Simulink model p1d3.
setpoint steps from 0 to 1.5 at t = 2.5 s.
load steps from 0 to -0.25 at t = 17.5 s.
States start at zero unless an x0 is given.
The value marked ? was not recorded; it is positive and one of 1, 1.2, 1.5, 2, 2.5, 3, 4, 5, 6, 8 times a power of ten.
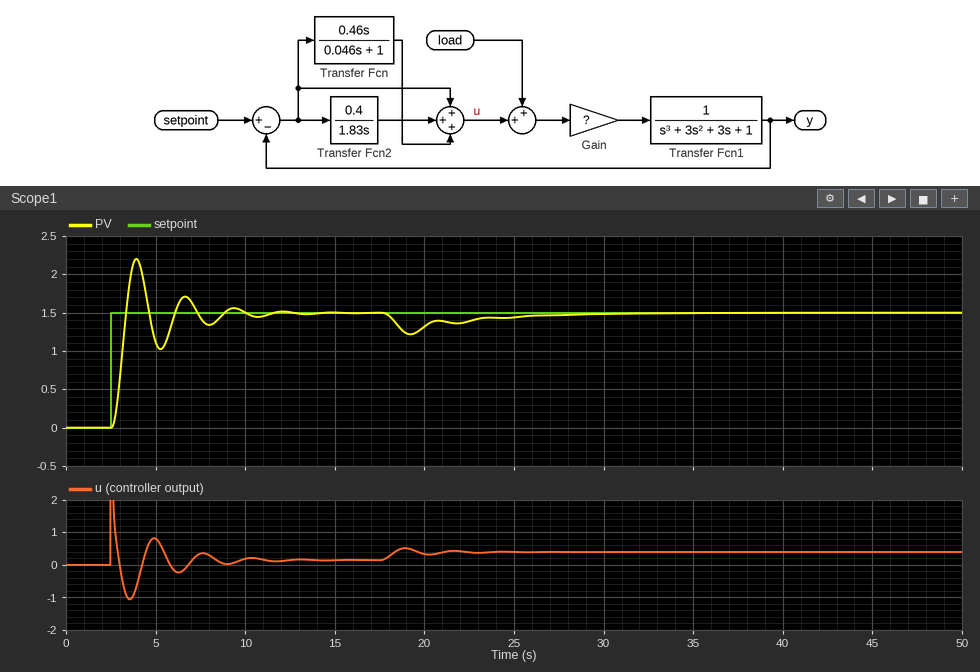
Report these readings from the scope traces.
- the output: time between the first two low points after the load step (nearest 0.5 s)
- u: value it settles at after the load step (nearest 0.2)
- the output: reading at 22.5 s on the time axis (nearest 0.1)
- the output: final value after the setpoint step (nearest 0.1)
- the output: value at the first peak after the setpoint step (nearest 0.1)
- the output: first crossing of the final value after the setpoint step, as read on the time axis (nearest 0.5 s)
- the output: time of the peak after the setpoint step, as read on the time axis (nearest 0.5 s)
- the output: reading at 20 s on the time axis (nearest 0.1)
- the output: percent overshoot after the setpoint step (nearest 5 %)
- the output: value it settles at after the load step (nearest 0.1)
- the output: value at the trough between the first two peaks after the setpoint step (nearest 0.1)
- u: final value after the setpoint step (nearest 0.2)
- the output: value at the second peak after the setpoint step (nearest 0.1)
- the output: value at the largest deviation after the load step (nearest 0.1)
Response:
2.5 s
0.4
1.4
1.5
2.2
3.5 s
4.0 s
1.3
45 %
1.5
1.0
0.2
1.7
1.2
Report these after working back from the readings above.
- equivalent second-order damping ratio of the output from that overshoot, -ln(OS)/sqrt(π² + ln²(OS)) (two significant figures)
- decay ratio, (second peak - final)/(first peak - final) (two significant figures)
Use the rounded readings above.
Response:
0.25
0.29
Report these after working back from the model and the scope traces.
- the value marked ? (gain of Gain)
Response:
10
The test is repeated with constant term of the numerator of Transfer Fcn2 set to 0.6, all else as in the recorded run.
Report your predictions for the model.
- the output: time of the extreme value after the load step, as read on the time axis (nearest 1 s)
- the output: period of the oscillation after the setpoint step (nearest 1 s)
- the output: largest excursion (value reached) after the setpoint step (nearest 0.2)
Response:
19 s
3 s
2.2
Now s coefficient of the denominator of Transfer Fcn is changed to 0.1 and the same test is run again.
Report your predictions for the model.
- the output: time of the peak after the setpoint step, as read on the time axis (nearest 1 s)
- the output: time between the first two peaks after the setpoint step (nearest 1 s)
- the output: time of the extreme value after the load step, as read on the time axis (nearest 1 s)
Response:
4 s
3 s
19 s
